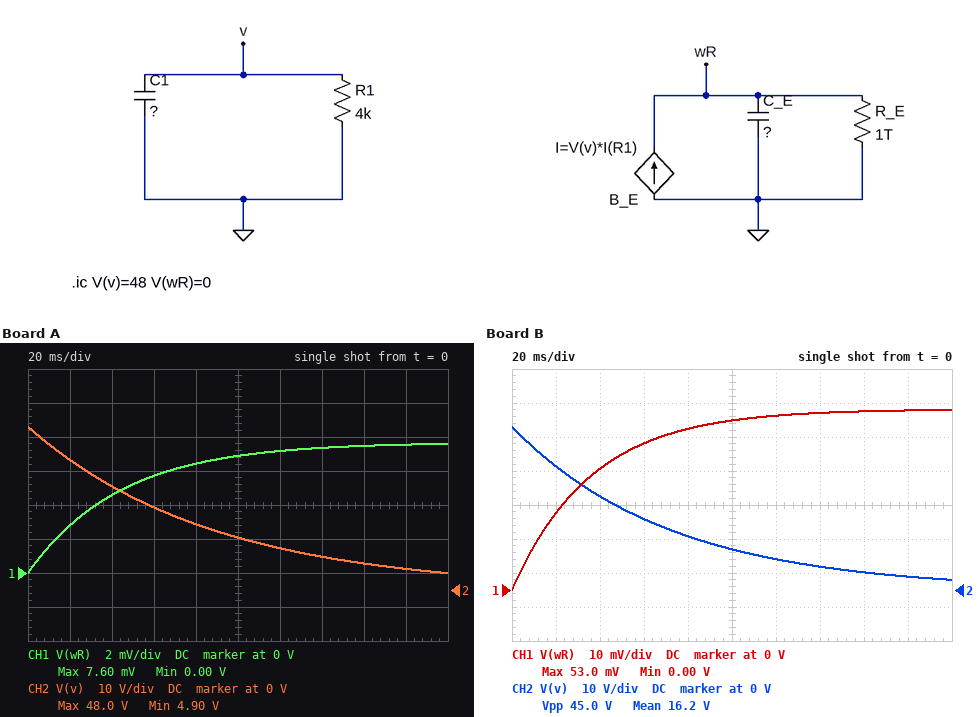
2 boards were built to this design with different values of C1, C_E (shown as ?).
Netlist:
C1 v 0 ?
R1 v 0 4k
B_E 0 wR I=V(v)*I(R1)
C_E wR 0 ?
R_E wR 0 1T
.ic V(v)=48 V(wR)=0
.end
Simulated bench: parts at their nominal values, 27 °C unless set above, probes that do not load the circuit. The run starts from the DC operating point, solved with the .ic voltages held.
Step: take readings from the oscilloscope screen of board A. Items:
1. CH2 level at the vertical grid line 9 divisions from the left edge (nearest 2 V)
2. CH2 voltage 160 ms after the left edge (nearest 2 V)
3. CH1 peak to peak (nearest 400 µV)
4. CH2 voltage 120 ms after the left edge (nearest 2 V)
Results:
6 V
8 V
7.6 mV
12 V
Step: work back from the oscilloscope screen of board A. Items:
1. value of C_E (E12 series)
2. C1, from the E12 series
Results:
3.3 F
22 µF
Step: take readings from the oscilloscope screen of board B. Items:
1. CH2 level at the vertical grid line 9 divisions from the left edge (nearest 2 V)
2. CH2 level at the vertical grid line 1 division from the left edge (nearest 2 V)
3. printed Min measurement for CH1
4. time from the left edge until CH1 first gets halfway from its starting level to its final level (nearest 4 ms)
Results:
4 V
36 V
0.00 V
24 ms
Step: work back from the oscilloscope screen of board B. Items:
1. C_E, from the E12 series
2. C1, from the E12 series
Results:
390 mF
18 µF
